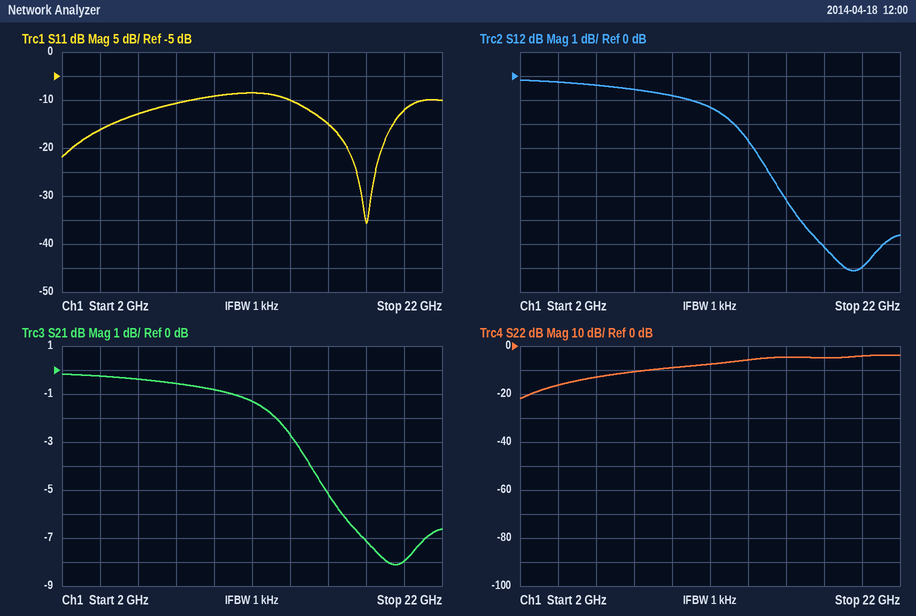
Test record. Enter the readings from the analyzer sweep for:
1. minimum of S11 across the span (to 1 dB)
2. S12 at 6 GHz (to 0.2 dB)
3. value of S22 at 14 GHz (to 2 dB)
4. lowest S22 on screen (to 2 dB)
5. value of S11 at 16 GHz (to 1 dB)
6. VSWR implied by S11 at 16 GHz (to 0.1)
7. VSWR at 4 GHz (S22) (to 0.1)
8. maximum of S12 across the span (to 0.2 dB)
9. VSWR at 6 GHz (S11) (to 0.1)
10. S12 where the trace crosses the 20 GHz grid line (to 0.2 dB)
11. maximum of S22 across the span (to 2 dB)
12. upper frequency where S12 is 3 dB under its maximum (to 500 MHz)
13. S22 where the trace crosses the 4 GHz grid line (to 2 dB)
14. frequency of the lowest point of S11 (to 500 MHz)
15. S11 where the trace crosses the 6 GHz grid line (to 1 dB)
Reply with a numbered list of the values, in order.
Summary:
1. -36 dB
2. -0.4 dB
3. -6 dB
4. -22 dB
5. -15 dB
6. 1.4
7. 1.4
8. -0.2 dB
9. 1.6
10. -8.0 dB
11. -4 dB
12. 14.5 GHz
13. -16 dB
14. 18.0 GHz
15. -13 dB
